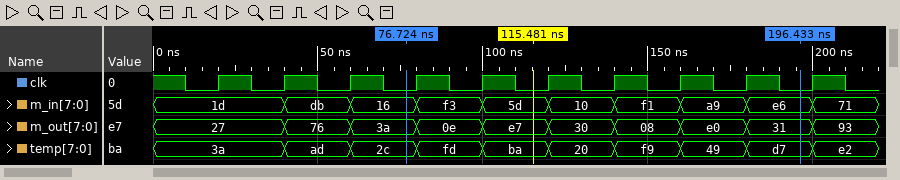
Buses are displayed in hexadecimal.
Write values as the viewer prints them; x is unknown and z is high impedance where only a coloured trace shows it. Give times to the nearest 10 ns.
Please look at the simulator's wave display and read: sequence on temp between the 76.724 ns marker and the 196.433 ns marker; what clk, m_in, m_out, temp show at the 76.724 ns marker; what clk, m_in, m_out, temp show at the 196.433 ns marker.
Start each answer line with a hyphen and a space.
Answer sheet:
- 2c, fd, ba, 20, f9, 49, d7
- clk=0, m_in=16, m_out=3a, temp=2c
- clk=0, m_in=e6, m_out=31, temp=d7
